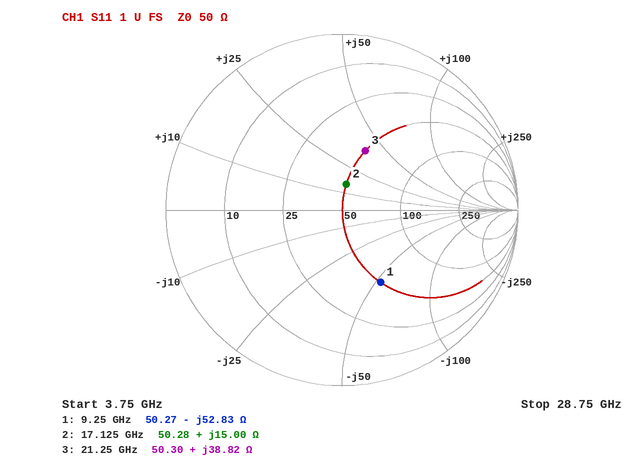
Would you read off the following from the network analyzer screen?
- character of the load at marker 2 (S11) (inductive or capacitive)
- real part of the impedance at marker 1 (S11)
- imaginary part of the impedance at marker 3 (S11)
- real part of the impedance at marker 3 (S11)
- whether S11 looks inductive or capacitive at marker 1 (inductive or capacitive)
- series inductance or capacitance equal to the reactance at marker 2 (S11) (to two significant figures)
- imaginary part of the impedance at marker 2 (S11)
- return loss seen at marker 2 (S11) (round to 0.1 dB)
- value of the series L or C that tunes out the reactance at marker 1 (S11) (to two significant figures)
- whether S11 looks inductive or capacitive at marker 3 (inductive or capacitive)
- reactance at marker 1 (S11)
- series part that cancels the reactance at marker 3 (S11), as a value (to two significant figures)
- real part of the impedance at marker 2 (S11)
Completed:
inductive
50.27 Ω
+38.82 Ω
50.30 Ω
capacitive
140 pH
+15.00 Ω
16.6 dB
910 pH
inductive
-52.83 Ω
190 fF
50.28 Ω
